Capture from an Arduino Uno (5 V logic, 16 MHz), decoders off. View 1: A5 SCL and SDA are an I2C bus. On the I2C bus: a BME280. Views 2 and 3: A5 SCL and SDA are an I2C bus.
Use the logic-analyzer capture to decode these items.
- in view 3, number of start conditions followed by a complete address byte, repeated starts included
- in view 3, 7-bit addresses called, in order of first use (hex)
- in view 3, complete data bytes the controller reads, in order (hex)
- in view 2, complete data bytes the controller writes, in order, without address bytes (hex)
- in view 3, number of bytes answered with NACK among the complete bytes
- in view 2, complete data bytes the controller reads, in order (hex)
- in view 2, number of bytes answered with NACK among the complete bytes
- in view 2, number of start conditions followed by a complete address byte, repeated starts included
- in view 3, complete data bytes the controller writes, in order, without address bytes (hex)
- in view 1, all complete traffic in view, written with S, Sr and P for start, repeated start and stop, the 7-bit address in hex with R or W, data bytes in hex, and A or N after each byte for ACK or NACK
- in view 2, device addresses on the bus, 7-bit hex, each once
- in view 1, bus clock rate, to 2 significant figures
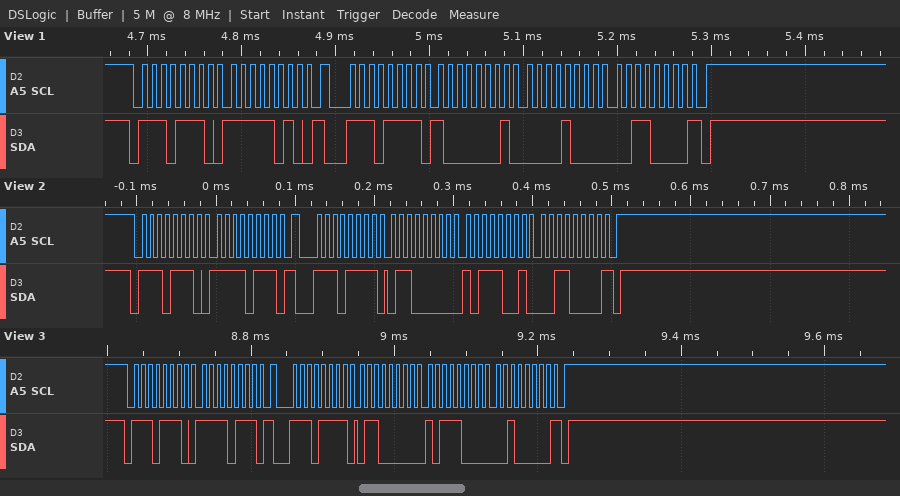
2
0x77
60 B8 20
F7
1
60 B9 30
1
2
F7
S 77W A FA A Sr 77R A 81 A 08 A 30 N P
0x77
100 kHz
